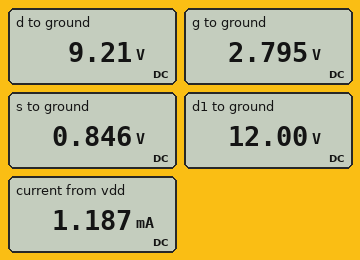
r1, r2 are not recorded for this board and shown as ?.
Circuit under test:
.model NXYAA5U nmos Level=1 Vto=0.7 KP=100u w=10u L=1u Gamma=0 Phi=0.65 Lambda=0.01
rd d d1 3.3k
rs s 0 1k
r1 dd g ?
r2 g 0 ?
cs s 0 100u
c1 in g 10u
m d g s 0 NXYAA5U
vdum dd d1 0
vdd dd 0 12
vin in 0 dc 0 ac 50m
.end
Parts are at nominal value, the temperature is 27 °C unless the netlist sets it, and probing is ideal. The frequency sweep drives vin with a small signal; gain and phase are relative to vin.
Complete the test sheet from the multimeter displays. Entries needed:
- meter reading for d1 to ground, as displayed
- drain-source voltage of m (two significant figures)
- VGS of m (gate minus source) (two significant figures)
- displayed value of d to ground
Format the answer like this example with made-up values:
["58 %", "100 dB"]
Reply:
["12.00 V", "8.4 V", "1.9 V", "9.21 V"]
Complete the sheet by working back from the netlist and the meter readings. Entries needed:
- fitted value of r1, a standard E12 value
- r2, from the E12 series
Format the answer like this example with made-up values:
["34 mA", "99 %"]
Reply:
["27 kΩ", "8.2 kΩ"]
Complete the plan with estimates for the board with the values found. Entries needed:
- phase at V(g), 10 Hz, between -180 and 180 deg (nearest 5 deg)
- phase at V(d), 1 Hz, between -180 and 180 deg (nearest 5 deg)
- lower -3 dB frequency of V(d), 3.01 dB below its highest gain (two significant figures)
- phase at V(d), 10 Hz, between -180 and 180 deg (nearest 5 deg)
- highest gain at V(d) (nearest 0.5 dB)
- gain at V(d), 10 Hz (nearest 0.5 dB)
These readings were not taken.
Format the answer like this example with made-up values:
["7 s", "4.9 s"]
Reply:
["15 deg", "-95 deg", "4.4 Hz", "-155 deg", "13.0 dB", "12.0 dB"]
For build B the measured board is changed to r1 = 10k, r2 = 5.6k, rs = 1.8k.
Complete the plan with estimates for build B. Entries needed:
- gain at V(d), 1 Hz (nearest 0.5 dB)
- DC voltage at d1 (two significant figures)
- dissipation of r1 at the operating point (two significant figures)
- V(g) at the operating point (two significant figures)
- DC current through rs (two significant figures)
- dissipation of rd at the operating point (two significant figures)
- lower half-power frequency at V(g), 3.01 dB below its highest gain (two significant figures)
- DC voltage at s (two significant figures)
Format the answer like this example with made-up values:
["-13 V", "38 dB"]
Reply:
["-7.5 dB", "12 V", "5.9 mW", "4.3 V", "1.2 mA", "4.6 mW", "4.4 Hz", "2.1 V"]
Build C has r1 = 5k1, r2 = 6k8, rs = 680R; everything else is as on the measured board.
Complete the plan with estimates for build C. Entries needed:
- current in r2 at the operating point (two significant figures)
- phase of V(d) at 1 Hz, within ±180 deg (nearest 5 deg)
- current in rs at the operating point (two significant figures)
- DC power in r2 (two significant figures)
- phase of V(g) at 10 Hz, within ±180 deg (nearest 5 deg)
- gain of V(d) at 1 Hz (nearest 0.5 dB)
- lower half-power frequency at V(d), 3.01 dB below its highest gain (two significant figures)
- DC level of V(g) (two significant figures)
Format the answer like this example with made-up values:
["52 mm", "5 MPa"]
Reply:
["1.0 mA", "-95 deg", "2.8 mA", "6.9 mW", "30 deg", "-31.0 dB", "5.9 Hz", "6.9 V"]
